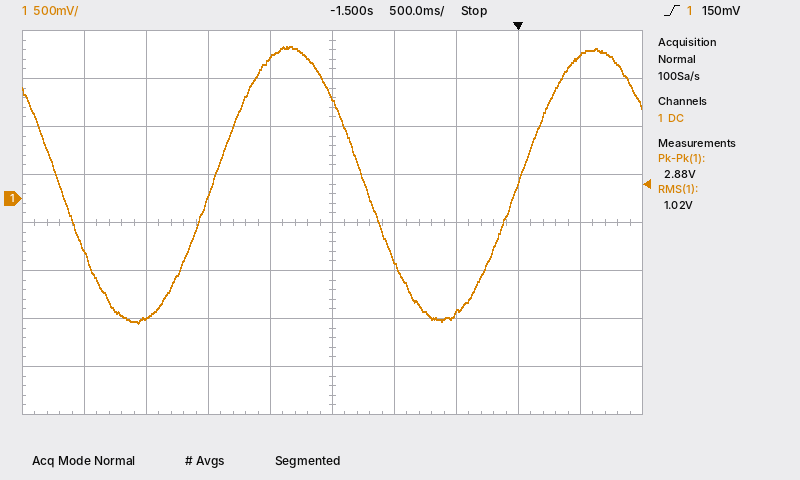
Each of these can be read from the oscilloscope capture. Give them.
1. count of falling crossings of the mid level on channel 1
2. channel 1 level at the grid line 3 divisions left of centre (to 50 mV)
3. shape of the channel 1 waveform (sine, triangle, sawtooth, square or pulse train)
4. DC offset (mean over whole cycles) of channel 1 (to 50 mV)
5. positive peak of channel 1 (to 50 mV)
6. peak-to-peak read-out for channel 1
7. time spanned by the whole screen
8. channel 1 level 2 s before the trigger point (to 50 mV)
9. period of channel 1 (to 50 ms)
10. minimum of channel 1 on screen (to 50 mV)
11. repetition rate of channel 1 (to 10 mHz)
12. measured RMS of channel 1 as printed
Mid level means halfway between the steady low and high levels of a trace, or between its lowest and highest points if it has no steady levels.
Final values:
2
-1.25 V
sine
150 mV
1.60 V
2.88 V
5 s
1.45 V
2.45 s
-1.30 V
410 mHz
1.02 V
